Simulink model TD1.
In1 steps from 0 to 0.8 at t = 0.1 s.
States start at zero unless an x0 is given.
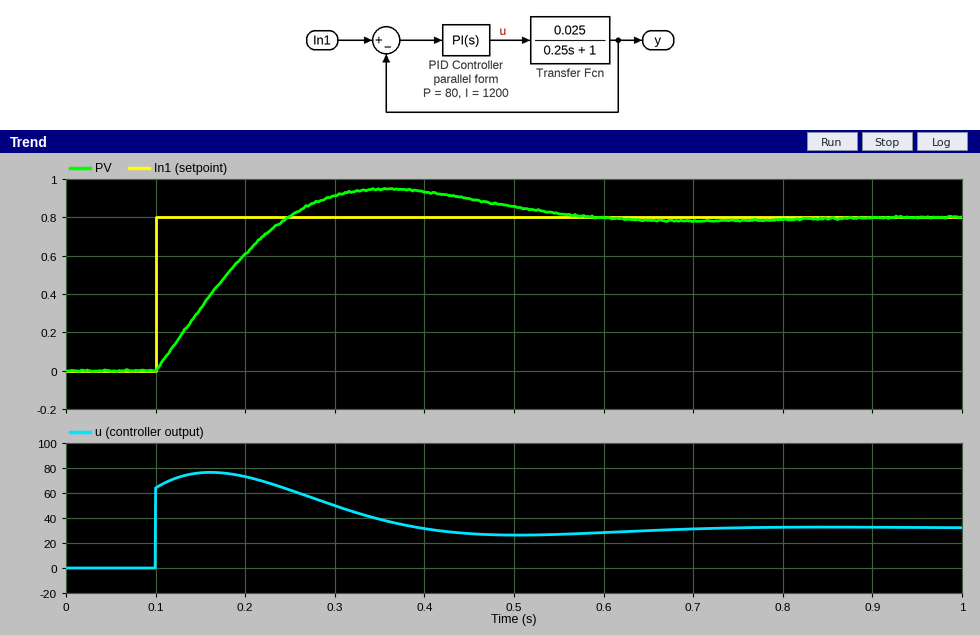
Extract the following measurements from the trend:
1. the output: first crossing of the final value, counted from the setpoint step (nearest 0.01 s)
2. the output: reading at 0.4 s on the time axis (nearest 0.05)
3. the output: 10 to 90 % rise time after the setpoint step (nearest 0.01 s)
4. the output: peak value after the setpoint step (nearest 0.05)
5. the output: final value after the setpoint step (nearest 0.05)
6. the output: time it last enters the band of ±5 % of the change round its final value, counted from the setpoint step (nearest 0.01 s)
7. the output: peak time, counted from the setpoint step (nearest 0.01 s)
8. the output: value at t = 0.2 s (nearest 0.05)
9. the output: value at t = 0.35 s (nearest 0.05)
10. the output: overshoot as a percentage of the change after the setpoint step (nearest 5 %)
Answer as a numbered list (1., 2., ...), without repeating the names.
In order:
1. 0.15 s
2. 0.95
3. 0.11 s
4. 0.95
5. 0.80
6. 0.42 s
7. 0.26 s
8. 0.60
9. 0.95
10. 20 %
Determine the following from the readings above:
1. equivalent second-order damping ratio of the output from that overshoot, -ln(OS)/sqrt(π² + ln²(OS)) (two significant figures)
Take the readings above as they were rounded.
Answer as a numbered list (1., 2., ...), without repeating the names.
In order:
1. 0.46
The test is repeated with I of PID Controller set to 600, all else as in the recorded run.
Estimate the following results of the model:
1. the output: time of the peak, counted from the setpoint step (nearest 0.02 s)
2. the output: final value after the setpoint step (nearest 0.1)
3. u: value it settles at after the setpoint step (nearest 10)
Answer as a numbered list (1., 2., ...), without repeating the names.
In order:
1. 0.38 s
2. 0.8
3. 30
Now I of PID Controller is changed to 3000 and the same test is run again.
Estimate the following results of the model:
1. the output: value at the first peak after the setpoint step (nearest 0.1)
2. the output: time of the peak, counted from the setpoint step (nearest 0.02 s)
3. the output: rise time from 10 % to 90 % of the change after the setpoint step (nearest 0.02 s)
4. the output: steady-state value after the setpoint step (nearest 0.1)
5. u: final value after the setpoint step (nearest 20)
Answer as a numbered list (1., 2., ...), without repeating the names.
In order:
1. 1.1
2. 0.16 s
3. 0.06 s
4. 0.8
5. 40
